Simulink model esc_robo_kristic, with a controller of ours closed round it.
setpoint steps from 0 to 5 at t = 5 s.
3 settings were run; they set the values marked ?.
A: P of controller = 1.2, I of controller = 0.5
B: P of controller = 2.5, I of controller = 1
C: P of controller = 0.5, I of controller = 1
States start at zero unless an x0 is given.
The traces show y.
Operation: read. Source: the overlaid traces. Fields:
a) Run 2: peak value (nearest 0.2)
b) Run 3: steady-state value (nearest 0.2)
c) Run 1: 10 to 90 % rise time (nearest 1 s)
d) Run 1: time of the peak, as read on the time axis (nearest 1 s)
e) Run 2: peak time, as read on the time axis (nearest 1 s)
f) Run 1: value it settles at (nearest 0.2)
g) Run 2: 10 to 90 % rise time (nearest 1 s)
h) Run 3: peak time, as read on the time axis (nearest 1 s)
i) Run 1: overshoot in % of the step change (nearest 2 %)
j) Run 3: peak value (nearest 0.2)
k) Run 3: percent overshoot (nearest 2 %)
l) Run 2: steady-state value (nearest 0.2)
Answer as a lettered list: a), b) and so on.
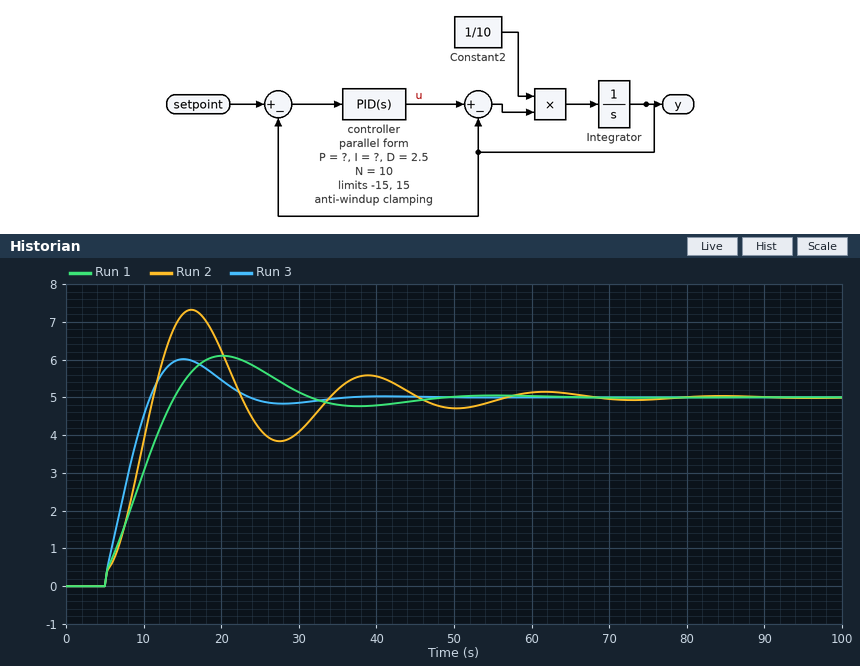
a) 7.4
b) 5.0
c) 7 s
d) 20 s
e) 16 s
f) 5.0
g) 5 s
h) 15 s
i) 22 %
j) 6.0
k) 20 %
l) 5.0
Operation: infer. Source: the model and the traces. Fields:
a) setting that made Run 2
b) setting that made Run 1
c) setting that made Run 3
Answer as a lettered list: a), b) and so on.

a) C
b) A
c) B
